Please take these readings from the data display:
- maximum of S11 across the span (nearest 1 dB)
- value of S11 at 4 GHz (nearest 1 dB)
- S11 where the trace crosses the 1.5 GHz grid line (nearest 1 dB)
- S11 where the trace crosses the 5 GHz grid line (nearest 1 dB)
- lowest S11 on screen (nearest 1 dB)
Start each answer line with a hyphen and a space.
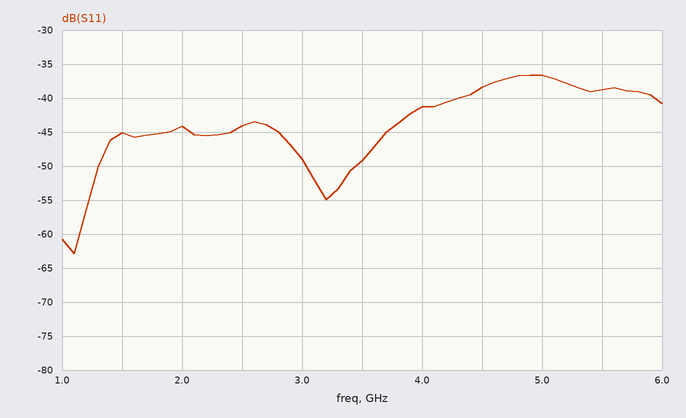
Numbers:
- -37 dB
- -41 dB
- -45 dB
- -37 dB
- -63 dB
